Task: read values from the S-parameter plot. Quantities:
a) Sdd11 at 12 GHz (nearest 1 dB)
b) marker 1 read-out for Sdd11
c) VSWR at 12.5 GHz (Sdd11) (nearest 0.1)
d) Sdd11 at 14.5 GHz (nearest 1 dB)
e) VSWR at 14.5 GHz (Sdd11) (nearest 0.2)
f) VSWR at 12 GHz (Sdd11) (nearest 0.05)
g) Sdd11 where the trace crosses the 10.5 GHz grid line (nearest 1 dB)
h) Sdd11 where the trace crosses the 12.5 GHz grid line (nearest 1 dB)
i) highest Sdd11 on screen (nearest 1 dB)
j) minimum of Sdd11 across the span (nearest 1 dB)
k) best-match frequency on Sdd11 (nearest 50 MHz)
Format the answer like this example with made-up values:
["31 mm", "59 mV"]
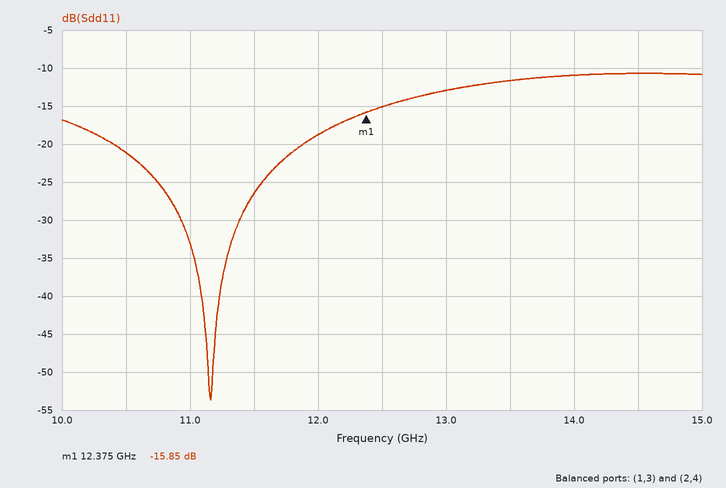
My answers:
["-19 dB", "-15.85 dB", "1.4", "-11 dB", "1.8", "1.25", "-21 dB", "-15 dB", "-11 dB", "-54 dB", "11.15 GHz"]
